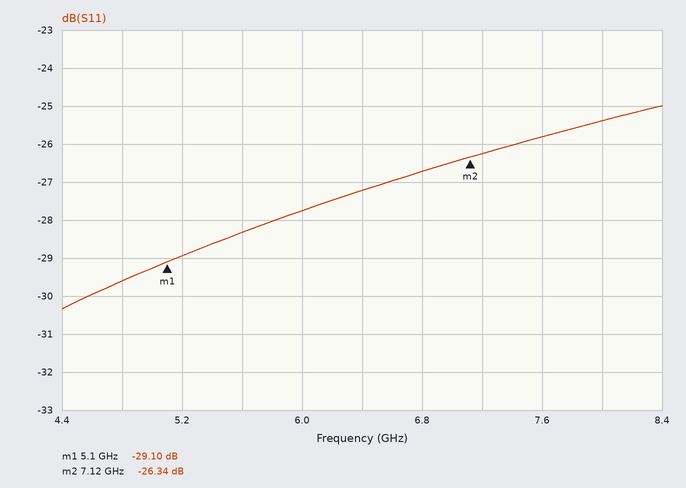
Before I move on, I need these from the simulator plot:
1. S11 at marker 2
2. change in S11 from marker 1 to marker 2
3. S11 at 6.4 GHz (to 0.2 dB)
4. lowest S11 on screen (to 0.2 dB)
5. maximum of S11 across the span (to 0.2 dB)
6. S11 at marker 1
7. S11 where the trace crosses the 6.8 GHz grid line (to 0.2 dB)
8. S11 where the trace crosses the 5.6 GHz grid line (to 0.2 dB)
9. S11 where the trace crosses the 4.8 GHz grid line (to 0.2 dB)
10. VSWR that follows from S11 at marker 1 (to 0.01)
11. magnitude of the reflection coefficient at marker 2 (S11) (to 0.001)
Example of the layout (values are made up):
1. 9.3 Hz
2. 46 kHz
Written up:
1. -26.34 dB
2. 2.76 dB
3. -27.2 dB
4. -30.4 dB
5. -25.0 dB
6. -29.10 dB
7. -26.8 dB
8. -28.4 dB
9. -29.6 dB
10. 1.07
11. 0.048
